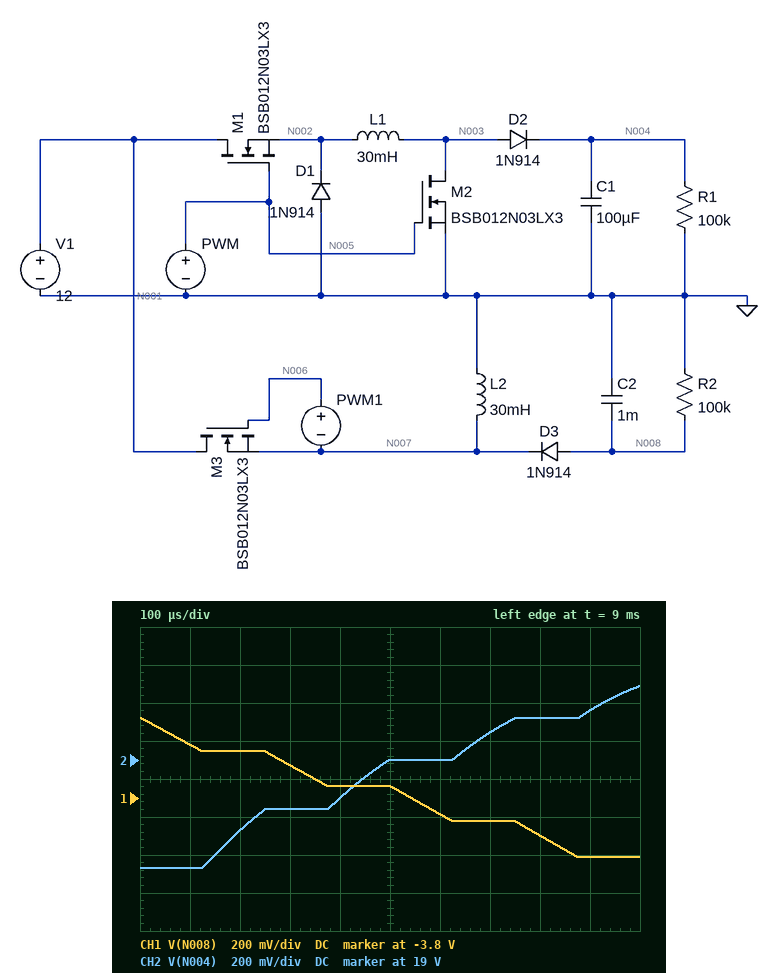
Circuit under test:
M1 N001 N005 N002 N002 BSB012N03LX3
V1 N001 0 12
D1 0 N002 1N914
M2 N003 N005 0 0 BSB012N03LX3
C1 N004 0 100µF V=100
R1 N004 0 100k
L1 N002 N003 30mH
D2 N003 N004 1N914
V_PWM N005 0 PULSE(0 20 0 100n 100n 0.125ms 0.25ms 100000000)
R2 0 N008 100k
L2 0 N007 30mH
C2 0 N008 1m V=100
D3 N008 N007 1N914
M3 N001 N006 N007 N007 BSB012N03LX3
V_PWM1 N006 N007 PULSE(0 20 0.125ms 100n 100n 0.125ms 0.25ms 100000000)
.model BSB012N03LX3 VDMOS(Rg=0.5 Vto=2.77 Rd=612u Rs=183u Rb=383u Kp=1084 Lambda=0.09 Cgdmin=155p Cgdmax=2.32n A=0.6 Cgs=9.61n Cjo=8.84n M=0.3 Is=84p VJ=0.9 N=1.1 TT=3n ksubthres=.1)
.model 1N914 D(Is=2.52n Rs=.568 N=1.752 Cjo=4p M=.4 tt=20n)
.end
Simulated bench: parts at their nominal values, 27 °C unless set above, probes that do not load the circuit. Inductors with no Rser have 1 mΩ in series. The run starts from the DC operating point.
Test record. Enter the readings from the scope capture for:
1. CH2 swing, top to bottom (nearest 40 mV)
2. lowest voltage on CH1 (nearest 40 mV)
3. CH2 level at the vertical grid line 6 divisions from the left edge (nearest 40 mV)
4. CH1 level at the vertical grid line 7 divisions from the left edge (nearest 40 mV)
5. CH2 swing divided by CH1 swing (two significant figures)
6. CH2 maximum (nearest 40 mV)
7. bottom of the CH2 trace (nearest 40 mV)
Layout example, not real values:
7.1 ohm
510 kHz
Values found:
960 mV
-4.12 V
19.00 V
-3.92 V
1.3
19.40 V
18.44 V
